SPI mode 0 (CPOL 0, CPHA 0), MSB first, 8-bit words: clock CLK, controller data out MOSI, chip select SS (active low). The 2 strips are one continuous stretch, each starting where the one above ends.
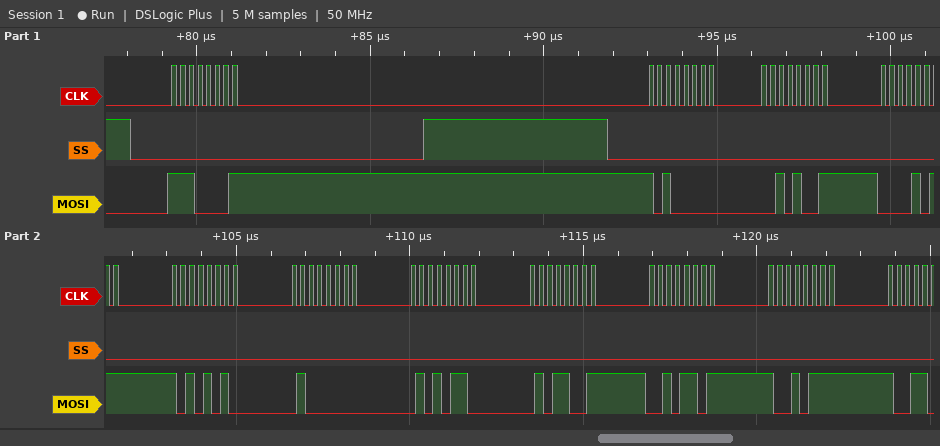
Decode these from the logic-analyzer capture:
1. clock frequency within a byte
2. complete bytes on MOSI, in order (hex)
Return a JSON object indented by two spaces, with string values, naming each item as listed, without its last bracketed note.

{
  "clock frequency within a byte": "4 MHz",
  "complete bytes on MOSI, in order": "E1 A0 29 0B AA 40 56 59 2D 97"
}
